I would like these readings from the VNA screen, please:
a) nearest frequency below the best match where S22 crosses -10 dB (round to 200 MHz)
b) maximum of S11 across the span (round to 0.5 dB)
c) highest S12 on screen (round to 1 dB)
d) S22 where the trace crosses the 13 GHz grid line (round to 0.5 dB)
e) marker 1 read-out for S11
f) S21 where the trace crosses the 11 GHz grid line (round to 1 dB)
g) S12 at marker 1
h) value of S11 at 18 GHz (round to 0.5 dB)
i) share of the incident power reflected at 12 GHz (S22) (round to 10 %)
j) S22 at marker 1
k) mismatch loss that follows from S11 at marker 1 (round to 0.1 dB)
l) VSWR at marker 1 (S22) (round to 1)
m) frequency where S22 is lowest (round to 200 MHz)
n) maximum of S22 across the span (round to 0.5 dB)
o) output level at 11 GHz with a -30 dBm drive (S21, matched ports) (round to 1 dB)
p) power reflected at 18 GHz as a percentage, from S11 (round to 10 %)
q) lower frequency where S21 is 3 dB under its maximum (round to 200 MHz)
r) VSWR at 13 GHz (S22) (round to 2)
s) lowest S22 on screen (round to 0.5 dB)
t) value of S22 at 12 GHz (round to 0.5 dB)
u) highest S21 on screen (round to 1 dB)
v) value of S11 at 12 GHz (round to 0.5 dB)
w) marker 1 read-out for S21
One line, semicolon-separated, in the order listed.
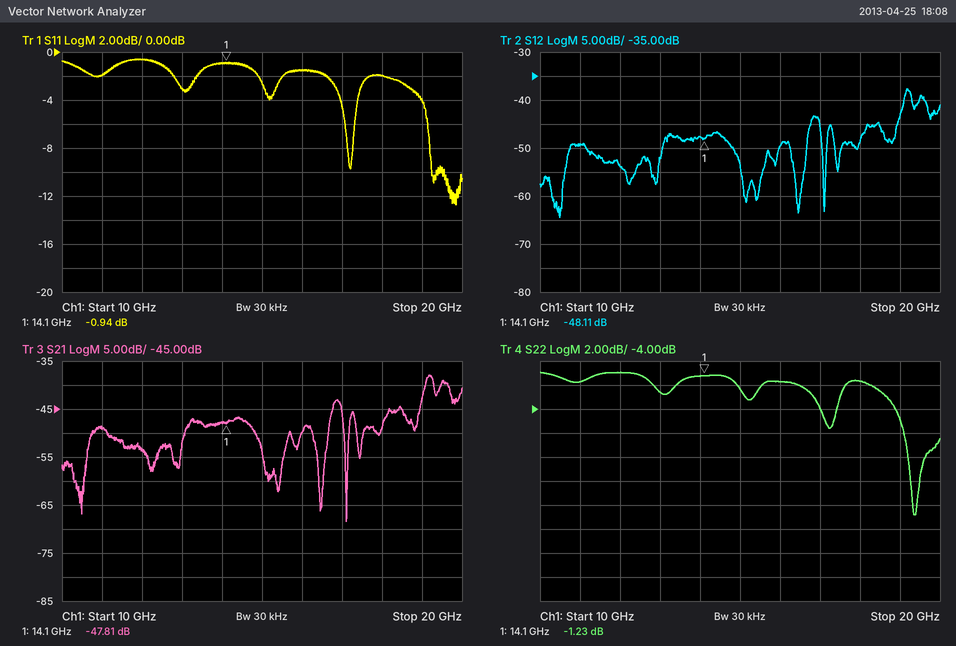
19.2 GHz; -0.5 dB; -38 dB; -2.5 dB; -0.94 dB; -49 dB; -48.11 dB; -2.0 dB; 80 %; -1.23 dB; 7.1 dB; 14; 19.4 GHz; -1.0 dB; -79 dBm; 60 %; 19.0 GHz; 6; -13.0 dB; -1.0 dB; -38 dB; -0.5 dB; -47.81 dB
